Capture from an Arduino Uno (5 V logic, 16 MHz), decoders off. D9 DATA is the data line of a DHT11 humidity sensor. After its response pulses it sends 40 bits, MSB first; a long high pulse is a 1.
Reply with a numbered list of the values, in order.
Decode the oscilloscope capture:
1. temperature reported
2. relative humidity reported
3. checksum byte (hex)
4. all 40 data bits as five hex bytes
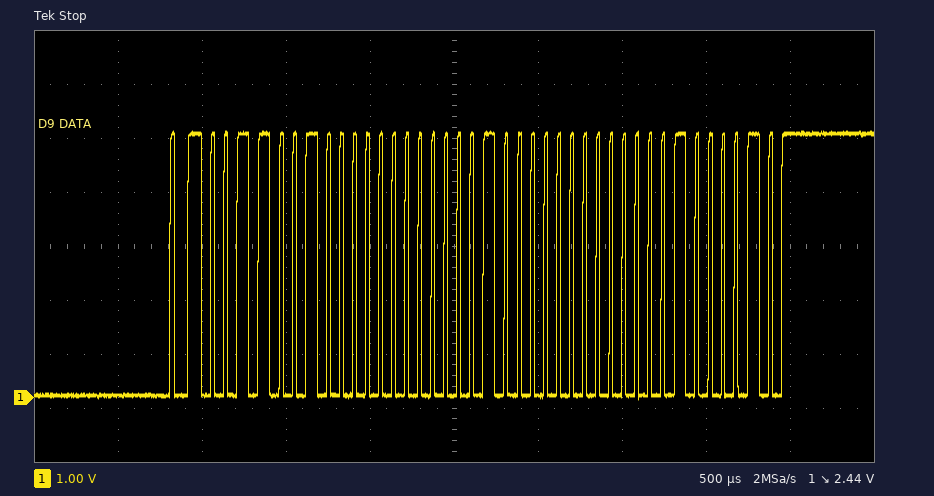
1. 16.0 °C
2. 50 %
3. 0x42
4. 32 00 10 00 42
